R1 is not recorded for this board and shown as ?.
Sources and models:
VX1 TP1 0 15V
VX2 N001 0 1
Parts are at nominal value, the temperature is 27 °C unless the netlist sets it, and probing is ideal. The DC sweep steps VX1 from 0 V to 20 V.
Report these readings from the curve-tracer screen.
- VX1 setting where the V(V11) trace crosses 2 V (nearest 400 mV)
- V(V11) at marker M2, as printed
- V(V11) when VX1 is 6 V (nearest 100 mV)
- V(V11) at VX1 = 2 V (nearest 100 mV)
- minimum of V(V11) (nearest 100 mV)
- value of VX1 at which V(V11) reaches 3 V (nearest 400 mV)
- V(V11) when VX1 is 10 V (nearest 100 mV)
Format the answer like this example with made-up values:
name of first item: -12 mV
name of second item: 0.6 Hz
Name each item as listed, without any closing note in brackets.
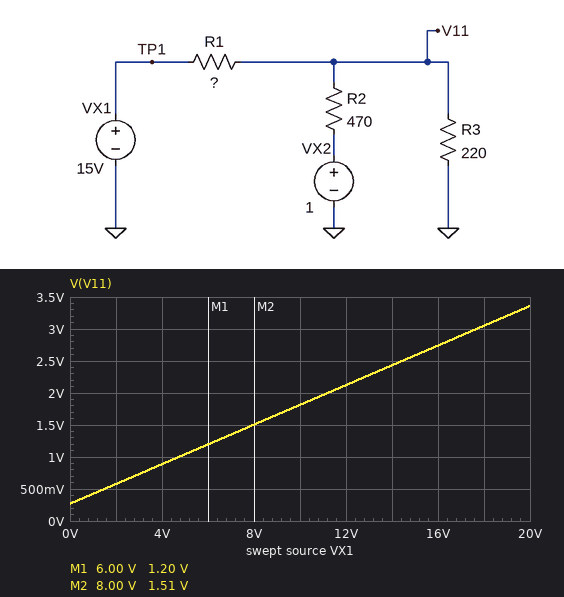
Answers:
VX1 setting where the V(V11) trace crosses 2 V: 11.2 V
V(V11) at marker M2, as printed: 1.51 V
V(V11) when VX1 is 6 V: 1.2 V
V(V11) at VX1 = 2 V: 600 mV
minimum of V(V11): 300 mV
value of VX1 at which V(V11) reaches 3 V: 17.6 V
V(V11) when VX1 is 10 V: 1.8 V
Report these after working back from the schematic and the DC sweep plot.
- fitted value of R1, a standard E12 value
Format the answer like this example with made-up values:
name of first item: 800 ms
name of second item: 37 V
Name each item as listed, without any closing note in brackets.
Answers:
fitted value of R1, a standard E12 value: 820 Ω
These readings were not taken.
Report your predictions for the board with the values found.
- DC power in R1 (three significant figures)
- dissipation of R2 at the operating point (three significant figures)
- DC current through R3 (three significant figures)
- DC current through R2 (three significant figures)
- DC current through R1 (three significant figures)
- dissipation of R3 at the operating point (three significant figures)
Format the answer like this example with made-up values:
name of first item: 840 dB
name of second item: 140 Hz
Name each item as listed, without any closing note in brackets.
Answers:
DC power in R1: 188 mW
dissipation of R2 at the operating point: 5.36 mW
DC current through R3: 11.8 mA
DC current through R2: 3.38 mA
DC current through R1: 15.1 mA
dissipation of R3 at the operating point: 30.4 mW
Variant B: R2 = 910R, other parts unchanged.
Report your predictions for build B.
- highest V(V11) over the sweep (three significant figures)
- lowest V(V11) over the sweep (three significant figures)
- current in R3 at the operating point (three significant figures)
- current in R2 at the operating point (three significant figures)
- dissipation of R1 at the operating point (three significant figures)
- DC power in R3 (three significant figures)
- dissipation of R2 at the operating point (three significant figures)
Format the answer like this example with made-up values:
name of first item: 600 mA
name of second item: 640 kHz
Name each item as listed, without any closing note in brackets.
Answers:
highest V(V11) over the sweep: 3.71 V
lowest V(V11) over the sweep: 160 mV
current in R3 at the operating point: 12.8 mA
current in R2 at the operating point: 2.01 mA
dissipation of R1 at the operating point: 181 mW
DC power in R3: 36.3 mW
dissipation of R2 at the operating point: 3.66 mW
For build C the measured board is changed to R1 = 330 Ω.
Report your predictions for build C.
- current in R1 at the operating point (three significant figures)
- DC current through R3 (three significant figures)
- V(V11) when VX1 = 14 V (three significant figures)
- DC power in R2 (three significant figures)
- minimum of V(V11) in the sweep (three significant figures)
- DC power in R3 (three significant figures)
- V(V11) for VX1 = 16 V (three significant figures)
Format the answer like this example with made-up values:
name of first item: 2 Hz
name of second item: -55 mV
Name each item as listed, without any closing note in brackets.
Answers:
current in R1 at the operating point: 30.6 mA
DC current through R3: 22.3 mA
V(V11) when VX1 = 14 V: 4.59 V
DC power in R2: 32.4 mW
minimum of V(V11) in the sweep: 219 mV
DC power in R3: 109 mW
V(V11) for VX1 = 16 V: 5.22 V
